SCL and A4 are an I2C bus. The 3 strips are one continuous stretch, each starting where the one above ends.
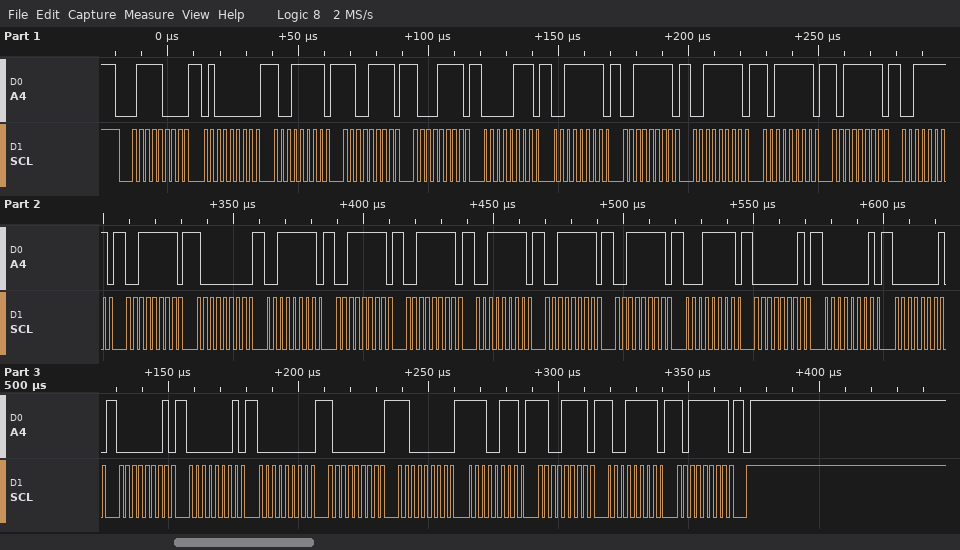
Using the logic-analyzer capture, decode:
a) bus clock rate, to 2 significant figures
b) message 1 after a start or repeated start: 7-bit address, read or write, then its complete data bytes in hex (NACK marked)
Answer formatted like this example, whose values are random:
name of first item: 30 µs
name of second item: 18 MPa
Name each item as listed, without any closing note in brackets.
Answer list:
bus clock rate, to 2 significant figures: 400 kHz
message 1 after a start or repeated start: 7-bit address, read or write, then its complete data bytes in hex: 0x3C write: 40 9F CF 8F 07 3F 3F 3F BF BF 3F 3F 80 3F 3F 3F 3F 3F 3F 1F 01 01 01 01 01 00 80 C0 E7 CF 9F BF
